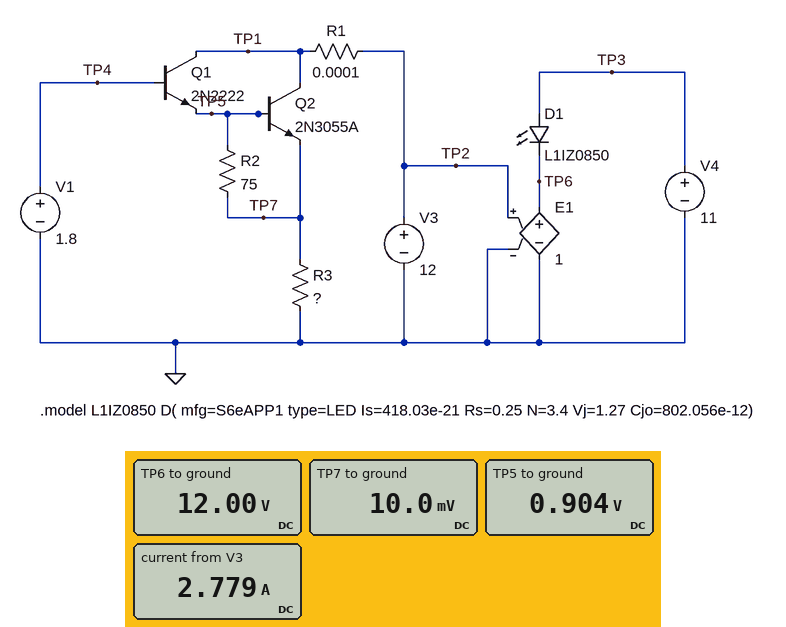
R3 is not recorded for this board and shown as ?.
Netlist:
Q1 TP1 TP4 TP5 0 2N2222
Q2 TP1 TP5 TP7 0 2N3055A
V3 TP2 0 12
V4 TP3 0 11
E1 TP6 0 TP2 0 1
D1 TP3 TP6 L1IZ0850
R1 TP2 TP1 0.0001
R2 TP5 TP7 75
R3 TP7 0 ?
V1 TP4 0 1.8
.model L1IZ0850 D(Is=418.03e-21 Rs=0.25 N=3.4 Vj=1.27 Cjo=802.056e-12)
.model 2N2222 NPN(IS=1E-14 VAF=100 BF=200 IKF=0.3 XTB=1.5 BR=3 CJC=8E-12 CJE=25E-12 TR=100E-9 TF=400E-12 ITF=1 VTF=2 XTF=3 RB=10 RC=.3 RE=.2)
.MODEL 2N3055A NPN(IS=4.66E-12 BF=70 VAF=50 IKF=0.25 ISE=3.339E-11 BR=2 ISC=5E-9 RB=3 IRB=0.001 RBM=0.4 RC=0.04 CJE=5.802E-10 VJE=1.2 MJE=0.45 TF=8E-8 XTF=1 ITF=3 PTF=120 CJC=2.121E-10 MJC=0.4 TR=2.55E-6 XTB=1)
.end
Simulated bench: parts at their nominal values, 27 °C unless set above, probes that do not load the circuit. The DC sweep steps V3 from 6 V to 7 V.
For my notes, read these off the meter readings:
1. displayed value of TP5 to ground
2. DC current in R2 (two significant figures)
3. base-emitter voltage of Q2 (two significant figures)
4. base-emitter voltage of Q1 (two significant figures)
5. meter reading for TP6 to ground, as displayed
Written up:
0.904 V
12 mA
890 mV
900 mV
12.00 V
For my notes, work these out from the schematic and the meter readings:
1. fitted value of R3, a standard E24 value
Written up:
3.6 mΩ
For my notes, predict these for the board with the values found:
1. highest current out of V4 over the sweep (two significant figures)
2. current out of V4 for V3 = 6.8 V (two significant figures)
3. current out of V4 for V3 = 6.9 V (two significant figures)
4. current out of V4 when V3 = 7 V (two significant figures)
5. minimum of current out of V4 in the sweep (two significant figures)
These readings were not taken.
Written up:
4.6 A
1.7 A
1.4 A
1.1 A
1.1 A
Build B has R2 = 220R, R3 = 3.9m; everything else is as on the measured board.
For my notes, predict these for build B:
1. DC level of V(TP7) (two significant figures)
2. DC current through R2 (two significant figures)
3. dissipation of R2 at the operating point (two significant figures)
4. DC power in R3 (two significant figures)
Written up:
11 mV
4.1 mA
3.6 mW
30 mW
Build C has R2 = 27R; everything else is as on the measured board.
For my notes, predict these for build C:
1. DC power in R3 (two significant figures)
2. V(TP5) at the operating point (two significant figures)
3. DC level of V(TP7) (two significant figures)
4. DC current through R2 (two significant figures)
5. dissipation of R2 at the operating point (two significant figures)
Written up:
27 mW
900 mV
9.9 mV
33 mA
29 mW
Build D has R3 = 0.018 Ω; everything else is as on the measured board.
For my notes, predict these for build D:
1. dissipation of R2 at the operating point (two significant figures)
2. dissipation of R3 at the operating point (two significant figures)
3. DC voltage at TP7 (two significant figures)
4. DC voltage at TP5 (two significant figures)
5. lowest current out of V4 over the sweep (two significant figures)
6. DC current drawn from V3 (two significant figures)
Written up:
10 mW
120 mW
46 mV
920 mV
1.1 A
2.6 A
